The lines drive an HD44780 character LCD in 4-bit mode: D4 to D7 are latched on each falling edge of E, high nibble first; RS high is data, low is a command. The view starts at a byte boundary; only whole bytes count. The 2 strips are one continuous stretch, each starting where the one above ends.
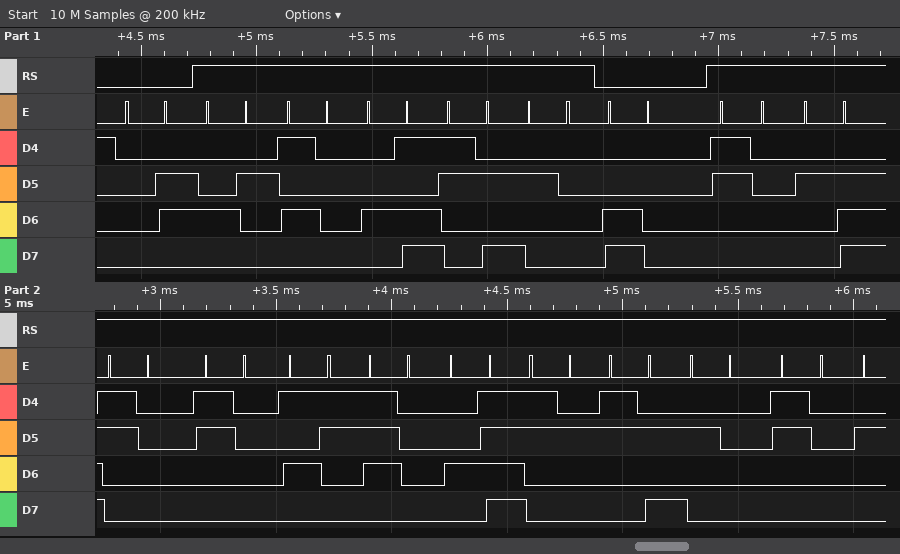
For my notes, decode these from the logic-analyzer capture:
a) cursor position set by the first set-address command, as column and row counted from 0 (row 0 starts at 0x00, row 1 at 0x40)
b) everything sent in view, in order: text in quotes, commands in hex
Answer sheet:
column 0, row 1
0x06 "BPM: " 0xC0 "0.00SpO2: 0"
